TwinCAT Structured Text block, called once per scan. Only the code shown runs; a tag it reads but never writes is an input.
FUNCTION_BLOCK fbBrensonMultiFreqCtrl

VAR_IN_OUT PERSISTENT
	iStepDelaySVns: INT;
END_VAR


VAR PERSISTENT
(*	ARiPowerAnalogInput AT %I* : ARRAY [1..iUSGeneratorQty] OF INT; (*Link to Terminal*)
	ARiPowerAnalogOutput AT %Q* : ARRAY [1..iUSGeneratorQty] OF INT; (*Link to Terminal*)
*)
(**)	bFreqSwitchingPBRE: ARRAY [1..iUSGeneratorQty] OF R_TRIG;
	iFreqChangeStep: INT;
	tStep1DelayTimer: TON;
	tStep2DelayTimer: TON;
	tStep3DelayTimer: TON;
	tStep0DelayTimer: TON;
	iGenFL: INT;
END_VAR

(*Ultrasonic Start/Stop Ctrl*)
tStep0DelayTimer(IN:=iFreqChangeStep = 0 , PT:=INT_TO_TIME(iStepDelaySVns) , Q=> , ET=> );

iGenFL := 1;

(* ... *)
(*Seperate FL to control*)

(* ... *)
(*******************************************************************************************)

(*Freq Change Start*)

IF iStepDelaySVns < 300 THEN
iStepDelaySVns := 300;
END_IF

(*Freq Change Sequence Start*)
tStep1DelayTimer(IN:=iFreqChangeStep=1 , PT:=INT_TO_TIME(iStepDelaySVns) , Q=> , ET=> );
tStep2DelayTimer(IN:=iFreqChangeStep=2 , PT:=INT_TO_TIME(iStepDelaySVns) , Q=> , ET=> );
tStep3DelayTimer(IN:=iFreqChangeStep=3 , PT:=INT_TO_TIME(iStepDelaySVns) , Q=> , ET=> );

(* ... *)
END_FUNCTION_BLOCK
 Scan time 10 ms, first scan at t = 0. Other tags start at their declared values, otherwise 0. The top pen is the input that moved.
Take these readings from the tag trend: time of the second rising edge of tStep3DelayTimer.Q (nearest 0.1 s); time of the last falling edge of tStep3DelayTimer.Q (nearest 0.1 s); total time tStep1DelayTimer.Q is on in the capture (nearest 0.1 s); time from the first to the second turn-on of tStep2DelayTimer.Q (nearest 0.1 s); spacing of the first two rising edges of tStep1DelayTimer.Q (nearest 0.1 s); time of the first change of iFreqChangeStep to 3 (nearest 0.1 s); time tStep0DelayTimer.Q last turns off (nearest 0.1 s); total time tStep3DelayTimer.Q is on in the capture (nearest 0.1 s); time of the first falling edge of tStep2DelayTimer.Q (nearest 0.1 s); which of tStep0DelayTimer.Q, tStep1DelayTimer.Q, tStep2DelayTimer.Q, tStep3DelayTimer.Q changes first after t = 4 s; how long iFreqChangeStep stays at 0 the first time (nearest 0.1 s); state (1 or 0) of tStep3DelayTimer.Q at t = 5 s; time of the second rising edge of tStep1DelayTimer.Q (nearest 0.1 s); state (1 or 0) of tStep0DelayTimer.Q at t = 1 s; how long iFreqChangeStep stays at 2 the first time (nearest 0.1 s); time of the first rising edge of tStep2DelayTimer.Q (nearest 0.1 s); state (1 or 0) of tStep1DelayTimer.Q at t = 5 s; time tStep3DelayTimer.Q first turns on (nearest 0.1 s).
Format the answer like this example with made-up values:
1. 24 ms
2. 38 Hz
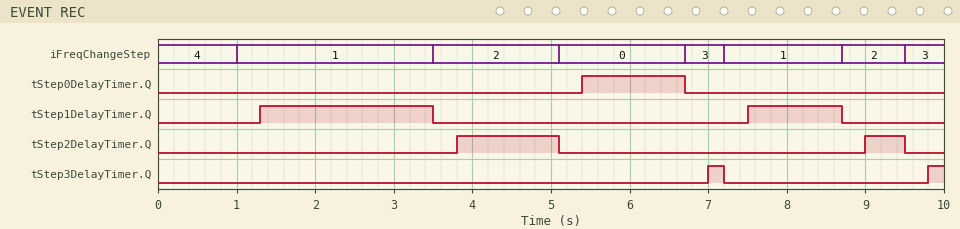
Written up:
1. 9.8 s
2. 7.2 s
3. 3.4 s
4. 5.2 s
5. 6.2 s
6. 6.7 s
7. 6.7 s
8. 0.4 s
9. 5.1 s
10. tStep2DelayTimer.Q
11. 1.6 s
12. 0
13. 7.5 s
14. 0
15. 1.6 s
16. 3.8 s
17. 0
18. 7.0 s
